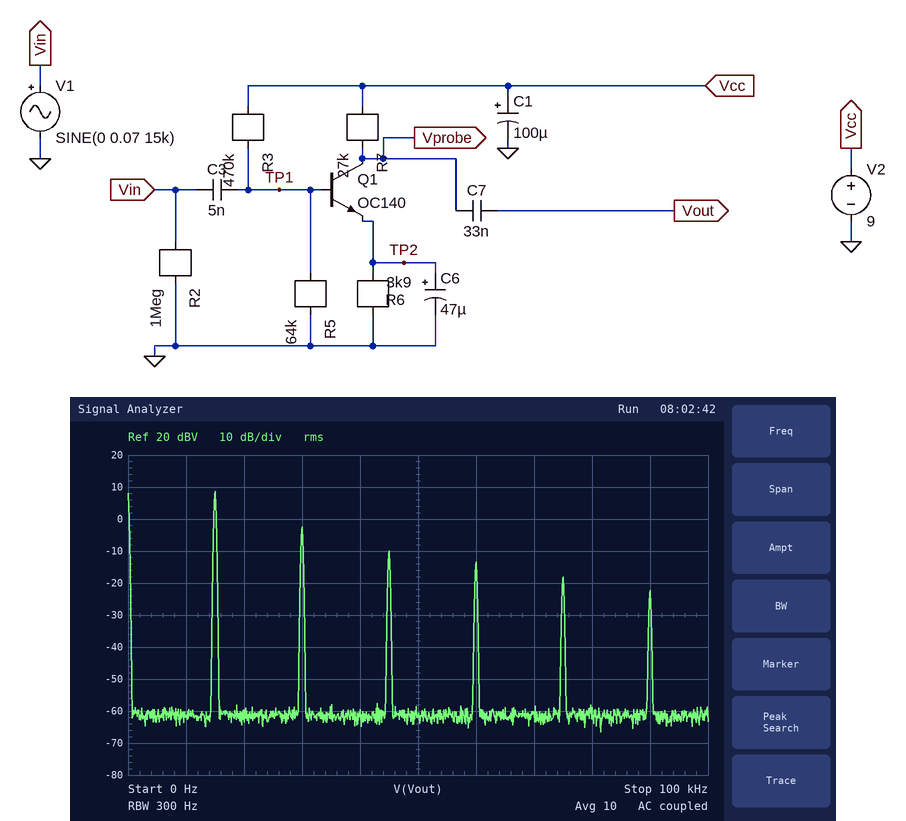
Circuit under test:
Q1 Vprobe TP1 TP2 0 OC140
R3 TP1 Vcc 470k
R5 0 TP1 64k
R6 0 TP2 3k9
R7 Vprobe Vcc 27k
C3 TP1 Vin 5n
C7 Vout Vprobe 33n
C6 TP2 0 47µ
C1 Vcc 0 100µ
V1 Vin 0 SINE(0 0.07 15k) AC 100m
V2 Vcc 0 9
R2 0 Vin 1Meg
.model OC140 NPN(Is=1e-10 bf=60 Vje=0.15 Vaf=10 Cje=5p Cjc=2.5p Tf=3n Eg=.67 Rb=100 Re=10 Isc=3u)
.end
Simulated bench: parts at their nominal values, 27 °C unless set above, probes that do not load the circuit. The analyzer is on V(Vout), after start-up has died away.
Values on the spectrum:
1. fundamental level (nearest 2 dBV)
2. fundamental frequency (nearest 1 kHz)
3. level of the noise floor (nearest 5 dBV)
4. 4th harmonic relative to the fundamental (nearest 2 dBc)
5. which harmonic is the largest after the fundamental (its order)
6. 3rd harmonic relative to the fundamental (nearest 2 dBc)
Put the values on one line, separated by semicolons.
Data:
8 dBV; 15 kHz; -60 dBV; -22 dBc; 2; -18 dBc
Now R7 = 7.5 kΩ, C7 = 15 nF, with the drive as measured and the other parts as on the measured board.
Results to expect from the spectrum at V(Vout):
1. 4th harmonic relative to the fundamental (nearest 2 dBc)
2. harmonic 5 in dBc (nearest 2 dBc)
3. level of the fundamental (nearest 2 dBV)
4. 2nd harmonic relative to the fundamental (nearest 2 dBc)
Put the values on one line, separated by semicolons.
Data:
-26 dBc; -32 dBc; 10 dBV; -22 dBc
